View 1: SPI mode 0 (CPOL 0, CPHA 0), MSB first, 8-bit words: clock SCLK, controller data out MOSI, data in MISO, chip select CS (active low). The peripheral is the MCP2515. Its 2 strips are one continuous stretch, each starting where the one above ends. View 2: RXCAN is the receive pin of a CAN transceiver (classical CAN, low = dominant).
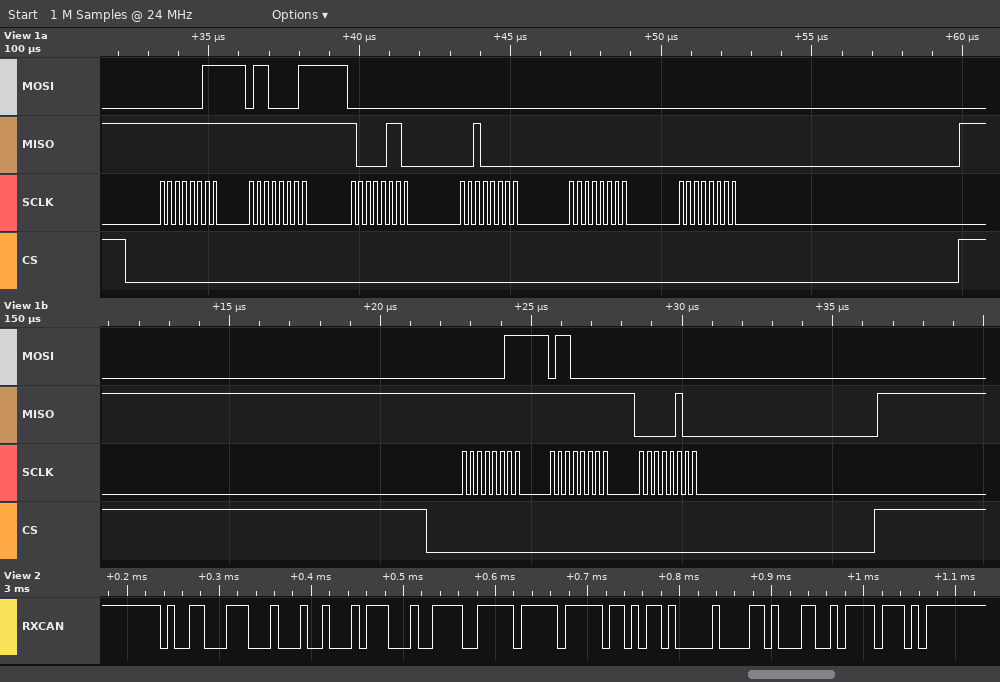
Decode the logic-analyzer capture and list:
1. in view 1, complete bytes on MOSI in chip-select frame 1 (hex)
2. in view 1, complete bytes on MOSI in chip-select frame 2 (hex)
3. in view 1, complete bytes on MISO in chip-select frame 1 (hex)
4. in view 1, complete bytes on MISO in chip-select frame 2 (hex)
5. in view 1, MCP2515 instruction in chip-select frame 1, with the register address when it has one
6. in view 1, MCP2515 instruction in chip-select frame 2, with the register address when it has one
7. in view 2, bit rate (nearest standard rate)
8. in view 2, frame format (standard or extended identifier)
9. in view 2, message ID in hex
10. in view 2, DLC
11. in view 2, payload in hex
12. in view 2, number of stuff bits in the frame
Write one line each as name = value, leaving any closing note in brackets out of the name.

in view 1, complete bytes on MOSI in chip-select frame 1 = 03 61 00 00 00 00
in view 1, complete bytes on MOSI in chip-select frame 2 = 03 60 00
in view 1, complete bytes on MISO in chip-select frame 1 = FF FF 86 20 00 00
in view 1, complete bytes on MISO in chip-select frame 2 = FF FF 04
in view 1, MCP2515 instruction in chip-select frame 1, with the register address when it has one = READ 0x61
in view 1, MCP2515 instruction in chip-select frame 2, with the register address when it has one = READ 0x60
in view 2, bit rate = 125 kbit/s
in view 2, frame format = standard
in view 2, message ID in hex = 0x4C7
in view 2, DLC = 8
in view 2, payload in hex = 91 71 3C FF FF AD 00 68
in view 2, number of stuff bits in the frame = 4
